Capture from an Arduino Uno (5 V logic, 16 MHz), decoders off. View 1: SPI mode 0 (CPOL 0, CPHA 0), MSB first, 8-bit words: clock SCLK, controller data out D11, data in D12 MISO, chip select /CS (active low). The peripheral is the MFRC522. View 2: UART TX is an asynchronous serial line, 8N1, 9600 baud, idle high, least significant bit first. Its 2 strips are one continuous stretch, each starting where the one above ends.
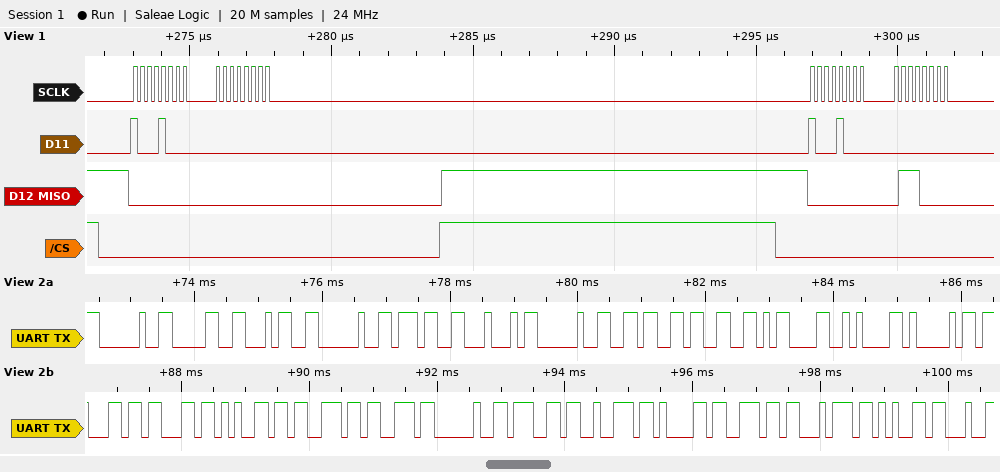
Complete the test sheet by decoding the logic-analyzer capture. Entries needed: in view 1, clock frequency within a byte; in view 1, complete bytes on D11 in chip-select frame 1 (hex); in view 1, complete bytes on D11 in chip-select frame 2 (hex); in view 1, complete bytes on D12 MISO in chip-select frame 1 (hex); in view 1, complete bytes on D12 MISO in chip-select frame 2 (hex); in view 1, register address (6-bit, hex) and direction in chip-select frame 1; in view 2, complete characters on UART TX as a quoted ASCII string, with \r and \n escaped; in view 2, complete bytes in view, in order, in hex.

4 MHz
88 00
88 00
00 00
00 70
0x04 read
" 04 7D 63\r\nAccess grante"
20 30 34 20 37 44 20 36 33 0D 0A 41 63 63 65 73 73 20 67 72 61 6E 74 65
